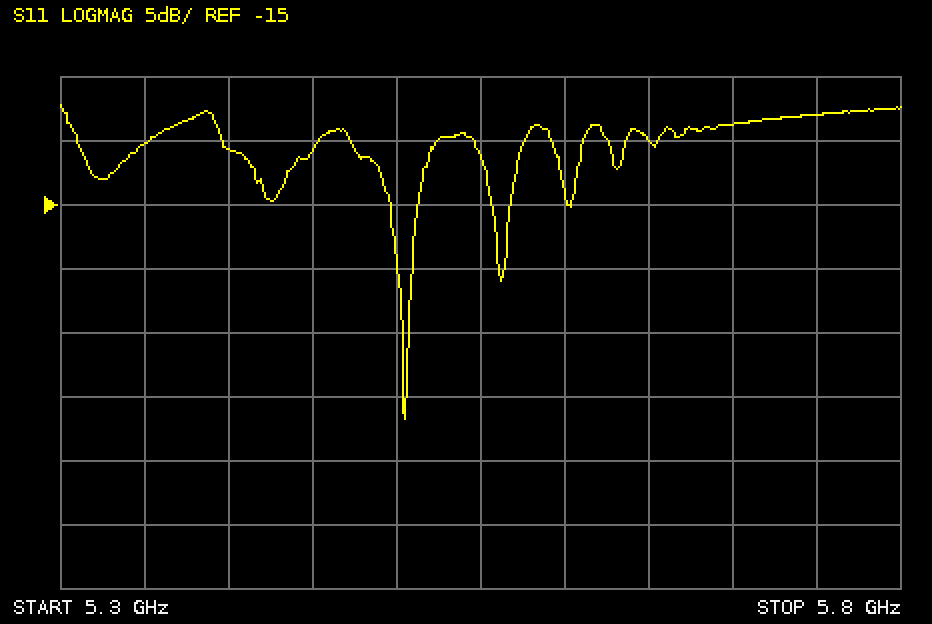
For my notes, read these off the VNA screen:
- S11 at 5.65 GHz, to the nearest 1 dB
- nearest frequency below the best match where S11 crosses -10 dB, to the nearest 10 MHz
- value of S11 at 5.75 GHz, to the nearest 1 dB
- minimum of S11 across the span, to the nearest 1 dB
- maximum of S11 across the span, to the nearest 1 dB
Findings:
-10 dB
5.47 GHz
-8 dB
-32 dB
-7 dB
